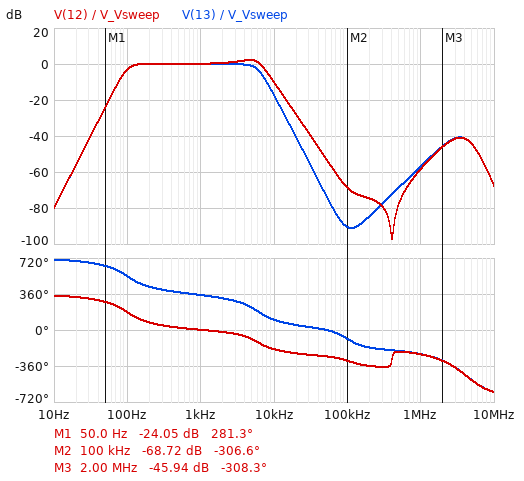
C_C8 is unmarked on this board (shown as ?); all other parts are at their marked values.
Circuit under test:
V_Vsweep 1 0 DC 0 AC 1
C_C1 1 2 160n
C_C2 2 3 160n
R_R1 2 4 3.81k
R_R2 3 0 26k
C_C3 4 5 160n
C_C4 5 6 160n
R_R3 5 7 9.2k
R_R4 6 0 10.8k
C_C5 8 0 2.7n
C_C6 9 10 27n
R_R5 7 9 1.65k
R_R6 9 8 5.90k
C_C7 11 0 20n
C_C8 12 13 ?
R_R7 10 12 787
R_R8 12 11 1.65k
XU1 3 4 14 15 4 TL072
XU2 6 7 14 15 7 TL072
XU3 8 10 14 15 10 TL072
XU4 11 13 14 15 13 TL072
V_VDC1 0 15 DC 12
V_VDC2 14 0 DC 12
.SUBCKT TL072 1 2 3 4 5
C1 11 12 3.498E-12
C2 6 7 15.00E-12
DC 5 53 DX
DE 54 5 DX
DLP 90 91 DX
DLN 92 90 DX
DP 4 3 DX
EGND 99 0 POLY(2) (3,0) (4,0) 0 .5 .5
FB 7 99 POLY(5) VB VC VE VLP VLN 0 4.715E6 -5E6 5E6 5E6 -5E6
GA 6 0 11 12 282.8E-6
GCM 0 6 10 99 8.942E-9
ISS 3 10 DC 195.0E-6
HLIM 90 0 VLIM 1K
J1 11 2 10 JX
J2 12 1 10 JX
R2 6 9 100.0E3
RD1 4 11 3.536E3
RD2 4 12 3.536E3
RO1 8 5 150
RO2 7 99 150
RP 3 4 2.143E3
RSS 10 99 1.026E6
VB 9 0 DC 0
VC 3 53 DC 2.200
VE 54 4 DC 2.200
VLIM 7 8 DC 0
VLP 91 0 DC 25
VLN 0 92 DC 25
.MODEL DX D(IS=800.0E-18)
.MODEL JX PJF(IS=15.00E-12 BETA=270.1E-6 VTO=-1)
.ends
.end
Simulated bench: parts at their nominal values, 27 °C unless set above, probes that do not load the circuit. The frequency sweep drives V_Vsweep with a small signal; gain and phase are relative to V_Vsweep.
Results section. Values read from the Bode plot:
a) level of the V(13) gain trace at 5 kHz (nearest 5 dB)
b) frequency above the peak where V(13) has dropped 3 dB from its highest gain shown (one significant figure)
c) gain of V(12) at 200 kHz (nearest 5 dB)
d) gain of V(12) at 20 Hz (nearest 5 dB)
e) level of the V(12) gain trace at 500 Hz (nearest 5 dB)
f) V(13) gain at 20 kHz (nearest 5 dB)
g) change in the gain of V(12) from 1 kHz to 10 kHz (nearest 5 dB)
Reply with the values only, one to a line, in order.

0 dB
6 kHz
-75 dB
-55 dB
0 dB
-40 dB
-10 dB
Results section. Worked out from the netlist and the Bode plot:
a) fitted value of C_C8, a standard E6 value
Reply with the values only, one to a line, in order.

22 nF
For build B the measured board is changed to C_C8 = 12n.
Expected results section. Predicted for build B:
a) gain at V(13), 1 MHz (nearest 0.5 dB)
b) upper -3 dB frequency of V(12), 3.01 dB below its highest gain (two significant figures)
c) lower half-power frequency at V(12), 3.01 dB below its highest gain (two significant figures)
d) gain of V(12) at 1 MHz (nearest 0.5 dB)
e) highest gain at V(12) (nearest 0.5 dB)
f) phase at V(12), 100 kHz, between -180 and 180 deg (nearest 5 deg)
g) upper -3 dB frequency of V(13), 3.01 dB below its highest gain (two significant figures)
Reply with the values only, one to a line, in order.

-57.0 dB
6.9 kHz
110 Hz
-60.0 dB
1.5 dB
60 deg
5.9 kHz
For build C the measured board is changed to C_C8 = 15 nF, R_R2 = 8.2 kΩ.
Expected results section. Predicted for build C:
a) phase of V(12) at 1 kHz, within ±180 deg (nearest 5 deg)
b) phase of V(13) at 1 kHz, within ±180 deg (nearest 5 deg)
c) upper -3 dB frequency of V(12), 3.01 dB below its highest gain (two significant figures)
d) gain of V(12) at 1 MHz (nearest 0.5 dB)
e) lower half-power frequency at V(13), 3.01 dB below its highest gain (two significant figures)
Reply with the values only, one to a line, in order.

10 deg
0 deg
6.9 kHz
-59.0 dB
200 Hz
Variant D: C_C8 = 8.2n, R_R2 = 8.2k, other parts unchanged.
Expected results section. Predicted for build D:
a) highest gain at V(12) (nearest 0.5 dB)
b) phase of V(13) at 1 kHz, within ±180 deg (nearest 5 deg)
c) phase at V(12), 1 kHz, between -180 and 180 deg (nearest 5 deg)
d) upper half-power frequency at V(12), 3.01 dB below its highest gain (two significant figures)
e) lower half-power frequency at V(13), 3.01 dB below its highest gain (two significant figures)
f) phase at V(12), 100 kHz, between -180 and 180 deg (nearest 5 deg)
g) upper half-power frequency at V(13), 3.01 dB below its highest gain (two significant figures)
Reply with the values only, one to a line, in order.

1.5 dB
0 deg
10 deg
6.9 kHz
200 Hz
65 deg
5.8 kHz
